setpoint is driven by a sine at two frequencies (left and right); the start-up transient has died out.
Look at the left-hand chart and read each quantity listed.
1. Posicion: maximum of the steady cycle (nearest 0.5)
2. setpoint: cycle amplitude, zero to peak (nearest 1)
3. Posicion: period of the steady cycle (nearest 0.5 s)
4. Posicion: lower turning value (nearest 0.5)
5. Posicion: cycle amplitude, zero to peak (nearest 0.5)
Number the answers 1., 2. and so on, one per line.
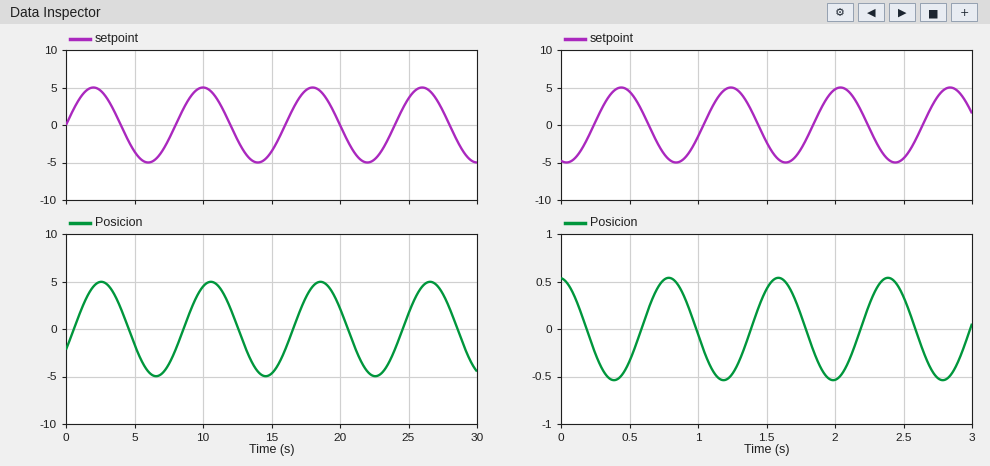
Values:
1. 5.0
2. 5
3. 8.0 s
4. -5.0
5. 5.0
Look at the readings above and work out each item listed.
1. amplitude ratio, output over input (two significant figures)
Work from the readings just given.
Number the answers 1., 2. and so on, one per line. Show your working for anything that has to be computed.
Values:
1. 5 / 5 = 1.0
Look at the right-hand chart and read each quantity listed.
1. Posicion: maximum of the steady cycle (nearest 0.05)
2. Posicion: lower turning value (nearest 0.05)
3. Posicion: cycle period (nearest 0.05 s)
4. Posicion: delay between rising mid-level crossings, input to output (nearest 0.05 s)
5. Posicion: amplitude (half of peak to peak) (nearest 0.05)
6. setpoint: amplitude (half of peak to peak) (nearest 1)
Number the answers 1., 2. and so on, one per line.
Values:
1. 0.55
2. -0.55
3. 0.80 s
4. 0.35 s
5. 0.55
6. 5
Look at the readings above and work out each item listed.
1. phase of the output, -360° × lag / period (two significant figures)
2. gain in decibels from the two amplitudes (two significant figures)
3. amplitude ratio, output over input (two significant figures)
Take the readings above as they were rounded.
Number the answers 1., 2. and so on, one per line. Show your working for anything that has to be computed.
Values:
1. -360 × 0.35 / 0.8 = -160°
2. 20 log10(0.55 / 5) = -19 dB
3. 0.55 / 5 = 0.11
